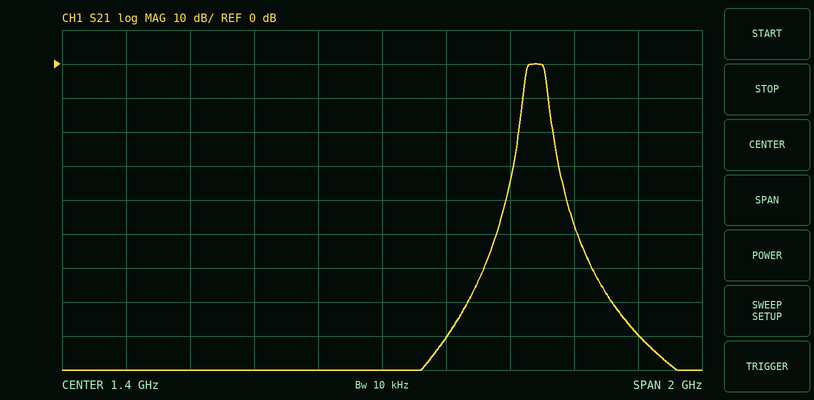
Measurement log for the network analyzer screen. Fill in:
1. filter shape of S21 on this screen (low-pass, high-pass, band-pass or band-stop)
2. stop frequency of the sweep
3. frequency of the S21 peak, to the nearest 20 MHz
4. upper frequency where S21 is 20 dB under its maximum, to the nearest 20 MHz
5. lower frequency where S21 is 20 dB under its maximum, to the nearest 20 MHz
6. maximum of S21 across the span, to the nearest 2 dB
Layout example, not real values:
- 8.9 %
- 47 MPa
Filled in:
- band-pass
- 2.4 GHz
- 1.88 GHz
- 1.94 GHz
- 1.82 GHz
- 0 dB
